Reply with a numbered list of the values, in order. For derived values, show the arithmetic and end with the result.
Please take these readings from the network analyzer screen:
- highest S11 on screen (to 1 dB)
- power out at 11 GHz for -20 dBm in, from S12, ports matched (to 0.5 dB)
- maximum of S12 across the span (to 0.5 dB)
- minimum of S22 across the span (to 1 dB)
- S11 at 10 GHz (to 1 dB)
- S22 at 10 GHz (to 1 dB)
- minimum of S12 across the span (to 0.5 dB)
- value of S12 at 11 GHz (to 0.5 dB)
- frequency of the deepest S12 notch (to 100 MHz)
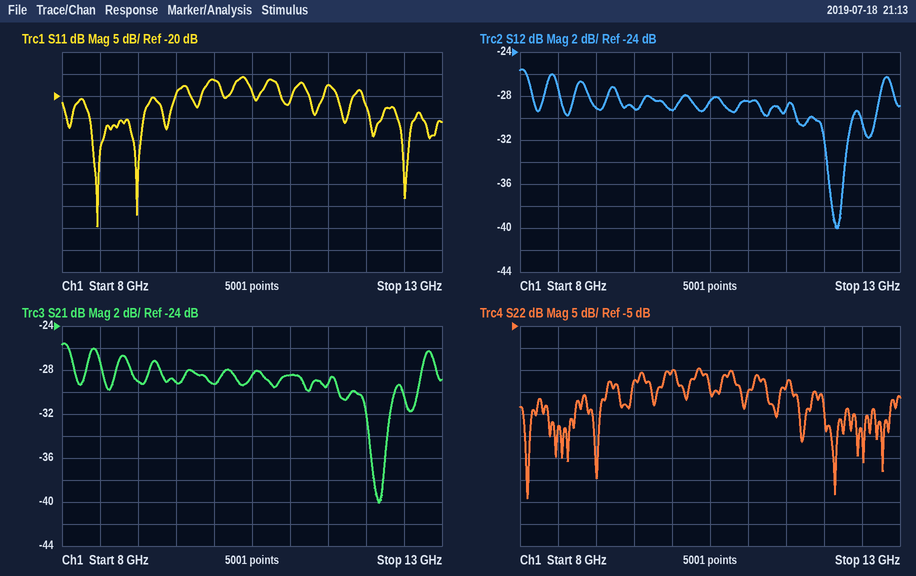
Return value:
1. -16 dB
2. -20 dBm + (-28.5 dB) = -48.5 dBm
3. -25.5 dB
4. -44 dB
5. -16 dB
6. -15 dB
7. -40.0 dB
8. -28.5 dB
9. 12.2 GHz
